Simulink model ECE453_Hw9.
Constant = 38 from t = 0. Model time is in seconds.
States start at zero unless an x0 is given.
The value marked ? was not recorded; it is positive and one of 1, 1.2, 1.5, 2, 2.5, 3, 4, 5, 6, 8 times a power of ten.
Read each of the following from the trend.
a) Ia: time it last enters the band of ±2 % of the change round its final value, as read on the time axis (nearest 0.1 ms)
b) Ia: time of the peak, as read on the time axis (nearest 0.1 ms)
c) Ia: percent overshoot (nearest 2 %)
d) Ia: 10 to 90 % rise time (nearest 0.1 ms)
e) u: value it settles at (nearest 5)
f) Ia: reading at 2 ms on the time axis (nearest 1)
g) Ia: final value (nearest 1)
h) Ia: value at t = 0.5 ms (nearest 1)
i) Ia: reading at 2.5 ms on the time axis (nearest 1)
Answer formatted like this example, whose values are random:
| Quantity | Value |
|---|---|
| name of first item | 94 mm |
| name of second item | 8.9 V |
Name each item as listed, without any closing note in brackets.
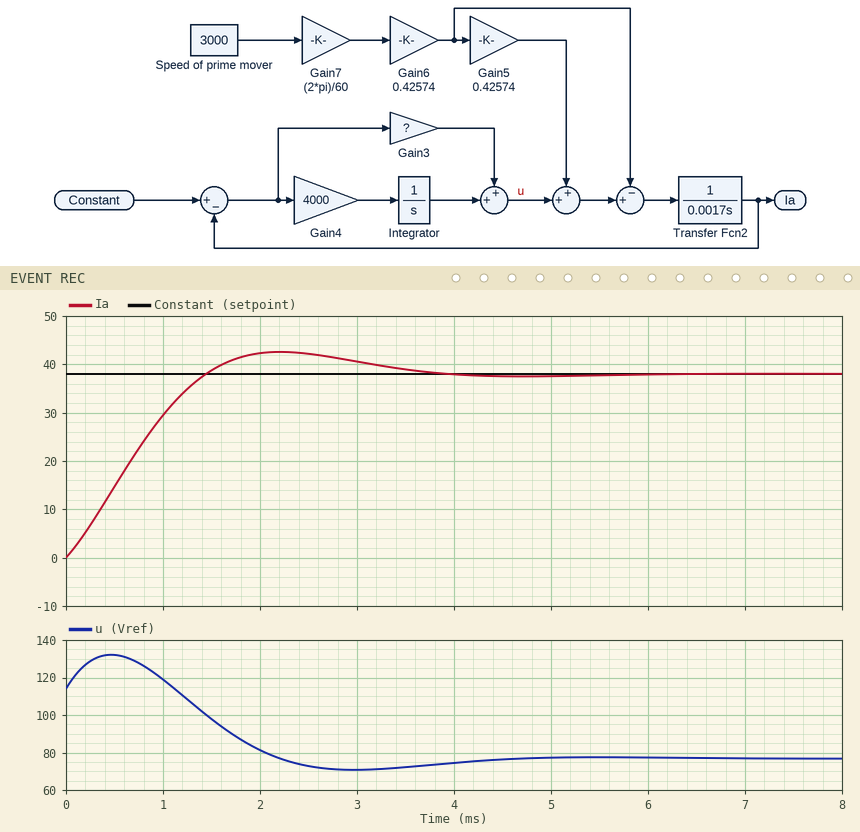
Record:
| Quantity | Value |
|---|---|
| Ia: time it last enters the band of ±2 % of the change round its final value, as read on the time axis | 3.6 ms |
| Ia: time of the peak, as read on the time axis | 2.2 ms |
| Ia: percent overshoot | 12 % |
| Ia: 10 to 90 % rise time | 1.1 ms |
| u: value it settles at | 75 |
| Ia: reading at 2 ms on the time axis | 42 |
| Ia: final value | 38 |
| Ia: value at t = 0.5 ms | 15 |
| Ia: reading at 2.5 ms on the time axis | 42 |
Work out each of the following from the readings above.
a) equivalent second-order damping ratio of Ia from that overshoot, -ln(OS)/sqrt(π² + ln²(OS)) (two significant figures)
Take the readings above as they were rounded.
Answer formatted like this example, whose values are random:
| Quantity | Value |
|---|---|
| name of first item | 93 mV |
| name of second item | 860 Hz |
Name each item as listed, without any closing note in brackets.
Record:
| Quantity | Value |
|---|---|
| equivalent second-order damping ratio of Ia from that overshoot, -ln(OS)/sqrt(π² + ln²(OS)) | 0.56 |
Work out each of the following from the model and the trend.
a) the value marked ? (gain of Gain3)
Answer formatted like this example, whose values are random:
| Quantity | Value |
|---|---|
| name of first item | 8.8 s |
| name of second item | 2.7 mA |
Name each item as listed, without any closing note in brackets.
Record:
| Quantity | Value |
|---|---|
| the value marked ? | 3 |
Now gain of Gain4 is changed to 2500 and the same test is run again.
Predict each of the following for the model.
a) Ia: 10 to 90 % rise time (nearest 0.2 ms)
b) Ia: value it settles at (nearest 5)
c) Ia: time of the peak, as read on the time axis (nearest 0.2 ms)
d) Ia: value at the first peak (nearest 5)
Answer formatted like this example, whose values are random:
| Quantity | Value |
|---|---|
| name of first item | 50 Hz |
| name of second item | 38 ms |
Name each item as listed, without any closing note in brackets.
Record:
| Quantity | Value |
|---|---|
| Ia: 10 to 90 % rise time | 1.6 ms |
| Ia: value it settles at | 40 |
| Ia: time of the peak, as read on the time axis | 3.2 ms |
| Ia: value at the first peak | 40 |
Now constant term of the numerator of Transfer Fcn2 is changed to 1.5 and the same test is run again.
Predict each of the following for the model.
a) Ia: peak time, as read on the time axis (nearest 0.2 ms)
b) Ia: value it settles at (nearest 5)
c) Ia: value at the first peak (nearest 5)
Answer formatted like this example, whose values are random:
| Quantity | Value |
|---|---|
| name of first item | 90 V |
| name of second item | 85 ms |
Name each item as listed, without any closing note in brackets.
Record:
| Quantity | Value |
|---|---|
| Ia: peak time, as read on the time axis | 2.0 ms |
| Ia: value it settles at | 40 |
| Ia: value at the first peak | 40 |
